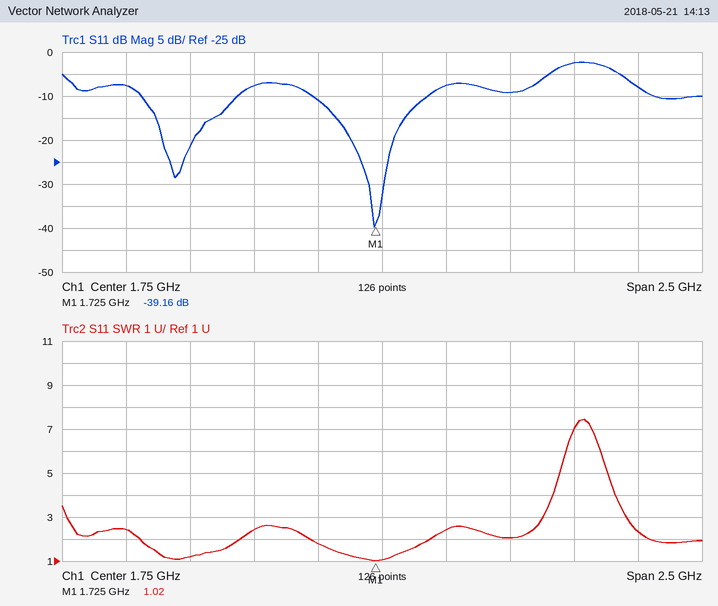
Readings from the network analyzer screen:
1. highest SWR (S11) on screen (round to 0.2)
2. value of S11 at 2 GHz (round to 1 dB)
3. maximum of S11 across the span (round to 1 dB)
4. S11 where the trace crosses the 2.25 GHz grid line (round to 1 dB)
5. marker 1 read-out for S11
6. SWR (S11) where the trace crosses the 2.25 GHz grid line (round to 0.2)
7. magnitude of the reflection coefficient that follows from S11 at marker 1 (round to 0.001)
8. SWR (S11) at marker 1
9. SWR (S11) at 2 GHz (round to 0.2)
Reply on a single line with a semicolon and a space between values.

7.4; -8 dB; -2 dB; -9 dB; -39.16 dB; 2.0; 0.011; 1.02; 2.4
